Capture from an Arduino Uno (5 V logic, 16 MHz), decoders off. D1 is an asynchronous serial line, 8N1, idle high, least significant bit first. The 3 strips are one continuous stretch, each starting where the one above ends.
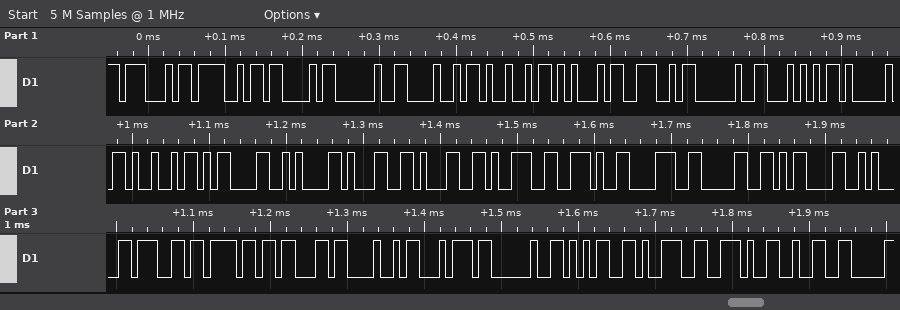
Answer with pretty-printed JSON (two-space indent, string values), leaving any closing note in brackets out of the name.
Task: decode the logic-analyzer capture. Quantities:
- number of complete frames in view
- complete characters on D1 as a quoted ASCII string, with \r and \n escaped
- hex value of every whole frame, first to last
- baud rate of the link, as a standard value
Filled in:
{
  "number of complete frames in view": "32",
  "complete characters on D1 as a quoted ASCII string, with \\r and \\n escaped": "\"GOC HIEN TAI\\r\\n119.80\\r\\ngocHt 59.2\"",
  "hex value of every whole frame, first to last": "47 4F 43 20 48 49 45 4E 20 54 41 49 0D 0A 31 31 39 2E 38 30 0D 0A 67 6F 63 48 74 20 35 39 2E 32",
  "baud rate of the link, as a standard value": "115200 baud"
}
